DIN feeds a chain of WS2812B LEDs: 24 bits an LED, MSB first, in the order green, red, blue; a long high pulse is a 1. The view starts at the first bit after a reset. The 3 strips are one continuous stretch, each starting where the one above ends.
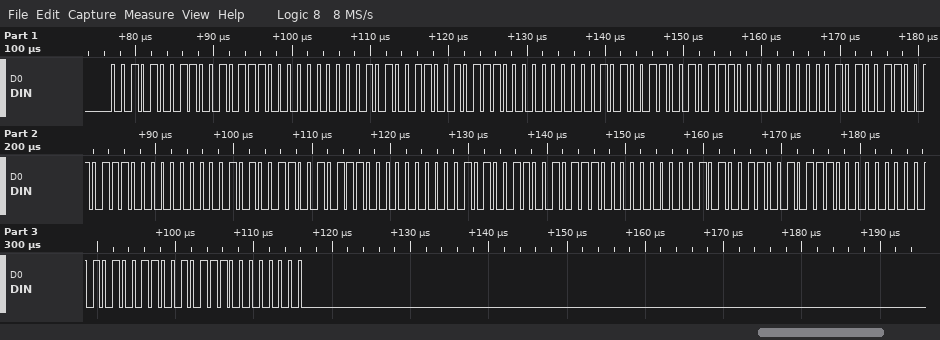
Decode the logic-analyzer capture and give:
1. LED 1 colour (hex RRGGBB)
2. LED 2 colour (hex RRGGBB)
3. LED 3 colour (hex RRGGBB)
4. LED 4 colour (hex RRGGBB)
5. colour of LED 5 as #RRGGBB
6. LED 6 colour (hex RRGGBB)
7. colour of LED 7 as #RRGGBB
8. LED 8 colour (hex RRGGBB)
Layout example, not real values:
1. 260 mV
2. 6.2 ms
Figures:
1. #972900
2. #972900
3. #972900
4. #972900
5. #972900
6. #972900
7. #972900
8. #972900
